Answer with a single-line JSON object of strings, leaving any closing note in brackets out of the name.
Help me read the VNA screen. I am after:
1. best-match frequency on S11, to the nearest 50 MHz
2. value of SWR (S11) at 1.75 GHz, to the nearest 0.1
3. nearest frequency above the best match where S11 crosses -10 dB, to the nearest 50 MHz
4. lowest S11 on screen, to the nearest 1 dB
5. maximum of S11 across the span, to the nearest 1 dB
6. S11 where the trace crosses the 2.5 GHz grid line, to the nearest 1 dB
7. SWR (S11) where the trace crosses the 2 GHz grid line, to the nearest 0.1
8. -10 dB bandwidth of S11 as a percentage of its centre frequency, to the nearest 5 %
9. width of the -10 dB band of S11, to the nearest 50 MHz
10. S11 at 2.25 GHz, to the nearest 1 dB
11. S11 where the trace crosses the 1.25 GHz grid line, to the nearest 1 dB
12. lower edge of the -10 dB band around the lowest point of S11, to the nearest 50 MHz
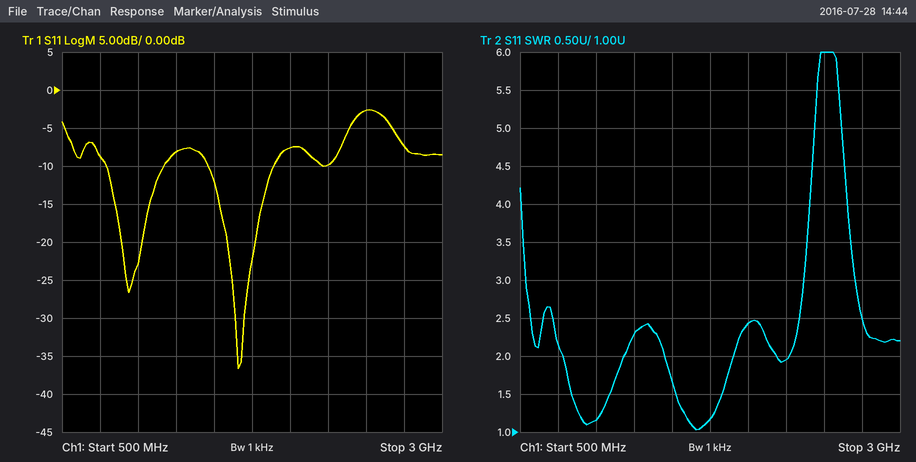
{"best-match frequency on S11, to the nearest 50 MHz": "1.65 GHz", "value of SWR (S11) at 1.75 GHz, to the nearest 0.1": "1.2", "nearest frequency above the best match where S11 crosses -10 dB, to the nearest 50 MHz": "1.90 GHz", "lowest S11 on screen, to the nearest 1 dB": "-37 dB", "maximum of S11 across the span, to the nearest 1 dB": "-3 dB", "S11 where the trace crosses the 2.5 GHz grid line, to the nearest 1 dB": "-3 dB", "SWR (S11) where the trace crosses the 2 GHz grid line, to the nearest 0.1": "2.4", "-10 dB bandwidth of S11 as a percentage of its centre frequency, to the nearest 5 %": "25 %", "width of the -10 dB band of S11, to the nearest 50 MHz": "450 MHz", "S11 at 2.25 GHz, to the nearest 1 dB": "-10 dB", "S11 where the trace crosses the 1.25 GHz grid line, to the nearest 1 dB": "-8 dB", "lower edge of the -10 dB band around the lowest point of S11, to the nearest 50 MHz": "1.45 GHz"}
